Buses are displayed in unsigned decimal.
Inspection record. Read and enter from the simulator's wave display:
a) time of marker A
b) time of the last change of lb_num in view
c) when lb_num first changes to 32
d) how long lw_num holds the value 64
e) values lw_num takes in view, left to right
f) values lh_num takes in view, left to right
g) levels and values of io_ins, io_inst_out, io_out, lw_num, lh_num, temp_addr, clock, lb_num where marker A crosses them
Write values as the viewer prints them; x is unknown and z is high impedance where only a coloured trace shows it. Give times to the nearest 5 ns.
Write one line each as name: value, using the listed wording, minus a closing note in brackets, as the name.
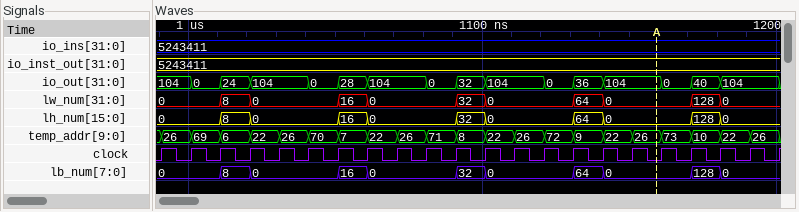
time of marker A: 1160 ns
time of the last change of lb_num in view: 1180 ns
when lb_num first changes to 32: 1090 ns
how long lw_num holds the value 64: 10 ns
values lw_num takes in view, left to right: 0, 8, 0, 16, 0, 32, 0, 64, 0, 128, 0
values lh_num takes in view, left to right: 0, 8, 0, 16, 0, 32, 0, 64, 0, 128, 0
levels and values of io_ins, io_inst_out, io_out, lw_num, lh_num, temp_addr, clock, lb_num where marker A crosses them: io_ins=5243411, io_inst_out=5243411, io_out=104, lw_num=0, lh_num=0, temp_addr=26, clock=0, lb_num=0
